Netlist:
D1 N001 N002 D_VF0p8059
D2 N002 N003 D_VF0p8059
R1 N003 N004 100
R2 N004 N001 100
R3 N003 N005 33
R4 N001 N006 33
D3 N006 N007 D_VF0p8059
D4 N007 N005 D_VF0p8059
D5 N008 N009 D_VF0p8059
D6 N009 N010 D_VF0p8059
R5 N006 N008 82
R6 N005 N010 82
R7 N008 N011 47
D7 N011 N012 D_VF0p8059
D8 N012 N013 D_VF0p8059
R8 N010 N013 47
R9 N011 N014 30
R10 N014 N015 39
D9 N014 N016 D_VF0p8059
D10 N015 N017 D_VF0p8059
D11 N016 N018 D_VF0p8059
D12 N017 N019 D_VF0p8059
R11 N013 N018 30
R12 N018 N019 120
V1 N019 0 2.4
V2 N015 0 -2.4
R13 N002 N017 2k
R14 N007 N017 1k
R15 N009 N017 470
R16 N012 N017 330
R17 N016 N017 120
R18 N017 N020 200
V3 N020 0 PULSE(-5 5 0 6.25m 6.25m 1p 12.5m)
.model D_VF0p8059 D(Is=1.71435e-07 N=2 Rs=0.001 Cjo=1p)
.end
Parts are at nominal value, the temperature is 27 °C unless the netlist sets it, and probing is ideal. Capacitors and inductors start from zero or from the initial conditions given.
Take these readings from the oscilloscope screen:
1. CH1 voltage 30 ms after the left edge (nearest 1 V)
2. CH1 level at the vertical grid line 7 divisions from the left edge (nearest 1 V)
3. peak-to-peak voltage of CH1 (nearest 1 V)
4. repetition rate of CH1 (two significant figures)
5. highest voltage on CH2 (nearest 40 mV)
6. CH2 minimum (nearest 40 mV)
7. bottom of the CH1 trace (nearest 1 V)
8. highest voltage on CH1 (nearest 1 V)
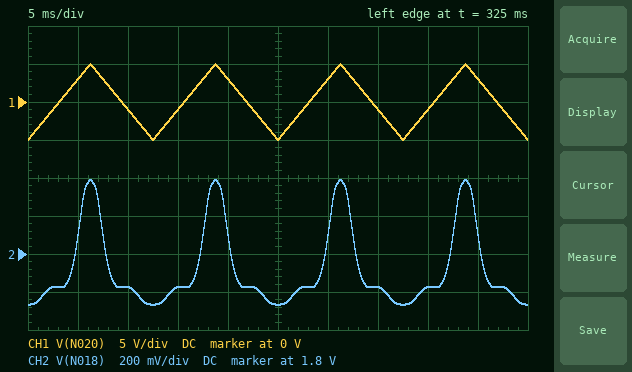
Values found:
3 V
-1 V
10 V
80 Hz
2.20 V
1.52 V
-5 V
5 V
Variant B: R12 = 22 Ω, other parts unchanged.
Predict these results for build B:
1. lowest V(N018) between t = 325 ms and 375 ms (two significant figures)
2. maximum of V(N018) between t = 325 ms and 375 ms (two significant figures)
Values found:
2.2 V
2.3 V
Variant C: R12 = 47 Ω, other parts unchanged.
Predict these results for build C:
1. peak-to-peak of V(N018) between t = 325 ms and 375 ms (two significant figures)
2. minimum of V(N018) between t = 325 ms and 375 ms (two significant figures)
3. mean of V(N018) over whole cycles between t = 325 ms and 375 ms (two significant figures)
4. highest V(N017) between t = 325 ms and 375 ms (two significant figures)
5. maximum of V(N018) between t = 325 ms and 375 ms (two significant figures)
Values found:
260 mV
2.0 V
2.1 V
2.9 V
2.3 V
